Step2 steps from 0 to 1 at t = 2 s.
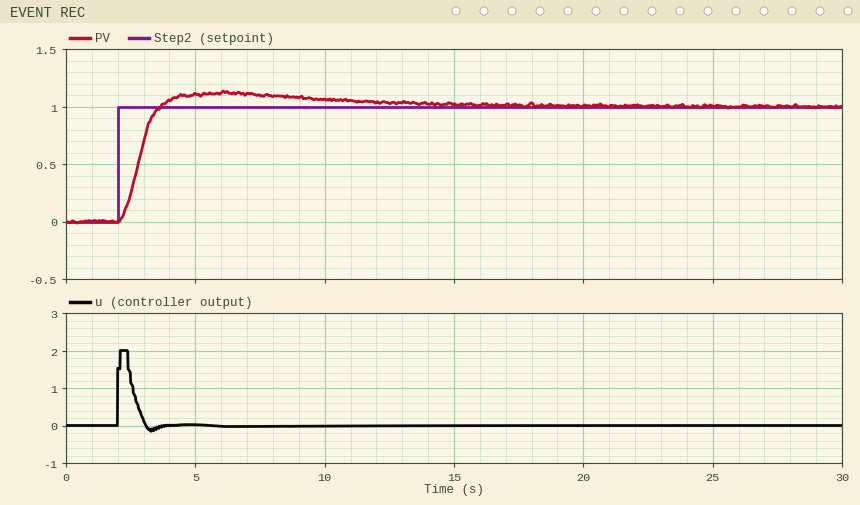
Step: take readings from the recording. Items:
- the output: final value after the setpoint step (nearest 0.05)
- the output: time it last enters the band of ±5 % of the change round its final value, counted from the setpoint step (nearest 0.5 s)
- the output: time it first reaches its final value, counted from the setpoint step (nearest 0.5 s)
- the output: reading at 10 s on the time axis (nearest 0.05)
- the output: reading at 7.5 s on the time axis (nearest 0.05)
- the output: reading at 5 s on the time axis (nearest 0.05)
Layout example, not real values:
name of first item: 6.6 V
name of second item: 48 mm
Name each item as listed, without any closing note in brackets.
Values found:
the output: final value after the setpoint step: 1.00
the output: time it last enters the band of ±5 % of the change round its final value, counted from the setpoint step: 9.0 s
the output: time it first reaches its final value, counted from the setpoint step: 1.5 s
the output: reading at 10 s on the time axis: 1.05
the output: reading at 7.5 s on the time axis: 1.10
the output: reading at 5 s on the time axis: 1.10
